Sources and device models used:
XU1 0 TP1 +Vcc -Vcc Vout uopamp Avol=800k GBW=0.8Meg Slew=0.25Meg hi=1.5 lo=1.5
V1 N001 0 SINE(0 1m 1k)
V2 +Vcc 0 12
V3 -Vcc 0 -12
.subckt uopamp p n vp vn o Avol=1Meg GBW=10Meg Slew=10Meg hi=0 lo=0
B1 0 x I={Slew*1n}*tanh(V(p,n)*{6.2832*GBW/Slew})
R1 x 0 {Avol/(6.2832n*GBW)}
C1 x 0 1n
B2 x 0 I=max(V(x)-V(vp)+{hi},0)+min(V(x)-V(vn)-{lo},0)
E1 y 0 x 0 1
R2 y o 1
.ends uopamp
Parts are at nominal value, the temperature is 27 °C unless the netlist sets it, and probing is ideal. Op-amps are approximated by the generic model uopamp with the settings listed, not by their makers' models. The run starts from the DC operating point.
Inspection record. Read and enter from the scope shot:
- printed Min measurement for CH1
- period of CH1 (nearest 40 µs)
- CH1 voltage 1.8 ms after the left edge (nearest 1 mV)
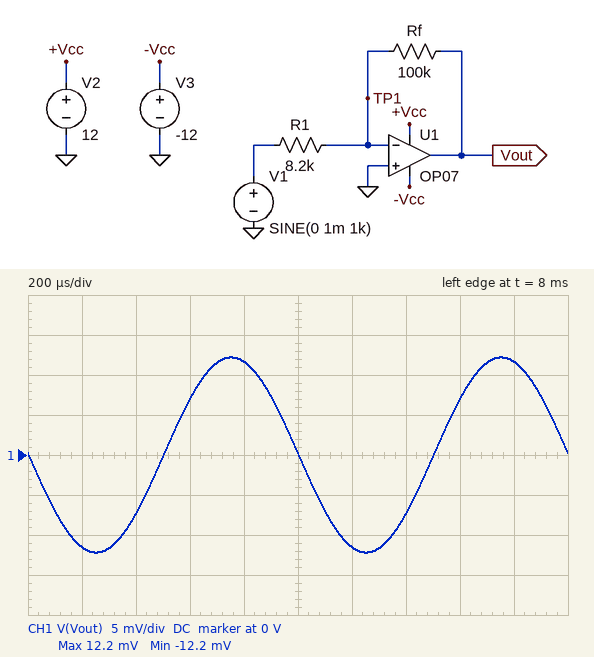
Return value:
-12.2 mV
1.00 ms
12 mV
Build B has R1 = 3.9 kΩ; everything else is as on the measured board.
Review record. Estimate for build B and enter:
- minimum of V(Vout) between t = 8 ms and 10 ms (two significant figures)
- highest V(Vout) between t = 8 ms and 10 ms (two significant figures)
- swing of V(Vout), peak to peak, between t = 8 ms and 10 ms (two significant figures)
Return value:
-26 mV
26 mV
51 mV
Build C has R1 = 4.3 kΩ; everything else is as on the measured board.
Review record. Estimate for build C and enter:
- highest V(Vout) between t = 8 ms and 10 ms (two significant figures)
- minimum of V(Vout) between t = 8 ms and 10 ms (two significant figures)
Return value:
23 mV
-23 mV
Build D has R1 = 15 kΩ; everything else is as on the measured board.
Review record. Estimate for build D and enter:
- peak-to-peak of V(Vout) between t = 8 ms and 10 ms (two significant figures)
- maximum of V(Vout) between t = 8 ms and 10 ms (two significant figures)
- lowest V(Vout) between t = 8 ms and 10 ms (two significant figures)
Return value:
13 mV
6.7 mV
-6.7 mV
